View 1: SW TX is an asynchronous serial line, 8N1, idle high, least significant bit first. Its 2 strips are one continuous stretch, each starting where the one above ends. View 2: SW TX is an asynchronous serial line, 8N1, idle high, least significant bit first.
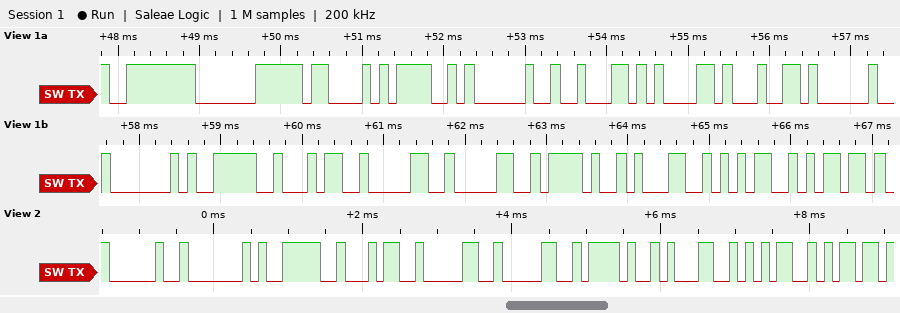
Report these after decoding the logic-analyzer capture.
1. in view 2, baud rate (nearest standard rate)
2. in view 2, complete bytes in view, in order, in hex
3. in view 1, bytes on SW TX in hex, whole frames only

9600 baud
0x20 0x40 0x3E 0x34 0x30 0x30 0x2F 0x31 0x35 0x6D
FE C0 43 4F 20 62 61 64 20 40 3E 34 30 30 2F 31 35 6D
